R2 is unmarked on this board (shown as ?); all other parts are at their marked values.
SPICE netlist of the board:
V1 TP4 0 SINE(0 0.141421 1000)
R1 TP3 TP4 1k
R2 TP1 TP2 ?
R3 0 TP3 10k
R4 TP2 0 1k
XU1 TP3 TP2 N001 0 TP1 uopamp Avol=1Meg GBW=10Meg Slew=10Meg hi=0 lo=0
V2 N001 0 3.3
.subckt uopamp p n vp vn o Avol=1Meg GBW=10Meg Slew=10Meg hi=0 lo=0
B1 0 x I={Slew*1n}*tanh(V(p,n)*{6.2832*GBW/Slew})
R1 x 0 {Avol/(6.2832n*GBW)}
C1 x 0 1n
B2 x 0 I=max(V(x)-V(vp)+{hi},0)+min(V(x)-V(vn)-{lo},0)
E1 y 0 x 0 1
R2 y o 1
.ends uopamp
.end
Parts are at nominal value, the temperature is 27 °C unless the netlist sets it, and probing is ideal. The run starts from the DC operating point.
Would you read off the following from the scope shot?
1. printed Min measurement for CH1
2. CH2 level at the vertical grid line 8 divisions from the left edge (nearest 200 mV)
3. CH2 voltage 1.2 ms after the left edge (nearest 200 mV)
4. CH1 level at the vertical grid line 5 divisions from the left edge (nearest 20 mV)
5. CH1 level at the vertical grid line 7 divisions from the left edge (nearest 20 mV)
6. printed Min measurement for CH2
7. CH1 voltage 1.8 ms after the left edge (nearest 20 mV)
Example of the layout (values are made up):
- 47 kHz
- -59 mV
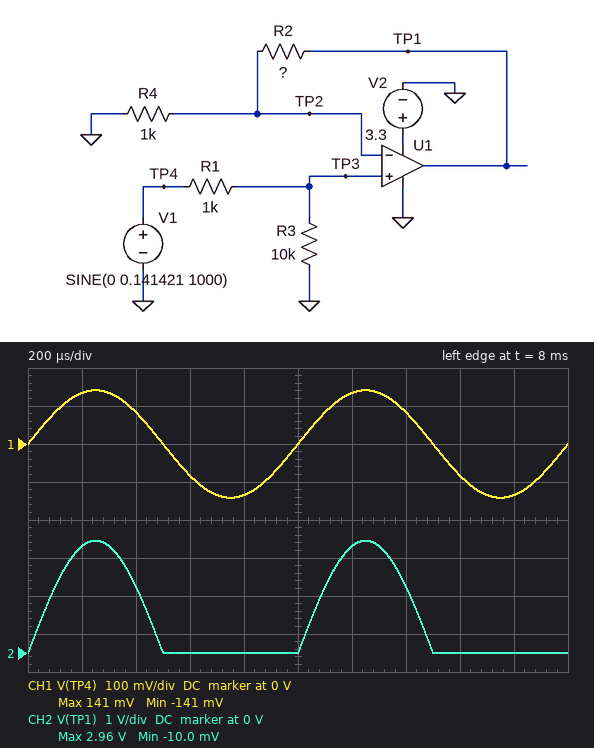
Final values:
- -141 mV
- 0 V
- 2.8 V
- 0 V
- 80 mV
- -10.0 mV
- -140 mV
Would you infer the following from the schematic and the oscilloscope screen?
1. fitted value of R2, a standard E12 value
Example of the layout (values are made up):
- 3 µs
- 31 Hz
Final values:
- 22 kΩ
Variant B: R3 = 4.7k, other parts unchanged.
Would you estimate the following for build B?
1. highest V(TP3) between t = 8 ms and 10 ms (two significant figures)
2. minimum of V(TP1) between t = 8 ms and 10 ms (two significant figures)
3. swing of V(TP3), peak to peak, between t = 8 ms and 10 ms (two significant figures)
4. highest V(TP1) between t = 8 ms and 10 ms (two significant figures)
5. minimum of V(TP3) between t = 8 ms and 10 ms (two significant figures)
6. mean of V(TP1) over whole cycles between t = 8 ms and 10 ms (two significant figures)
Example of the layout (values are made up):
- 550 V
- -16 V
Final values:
- 120 mV
- -6.2 mV
- 230 mV
- 2.7 V
- -120 mV
- 850 mV
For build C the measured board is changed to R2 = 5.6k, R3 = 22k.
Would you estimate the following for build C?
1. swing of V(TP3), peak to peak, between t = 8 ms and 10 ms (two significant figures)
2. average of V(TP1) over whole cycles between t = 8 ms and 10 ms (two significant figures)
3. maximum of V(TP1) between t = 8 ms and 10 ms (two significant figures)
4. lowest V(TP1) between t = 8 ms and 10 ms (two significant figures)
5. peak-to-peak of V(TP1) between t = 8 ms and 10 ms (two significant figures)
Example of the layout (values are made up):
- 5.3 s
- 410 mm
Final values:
- 270 mV
- 280 mV
- 890 mV
- -6.9 mV
- 900 mV
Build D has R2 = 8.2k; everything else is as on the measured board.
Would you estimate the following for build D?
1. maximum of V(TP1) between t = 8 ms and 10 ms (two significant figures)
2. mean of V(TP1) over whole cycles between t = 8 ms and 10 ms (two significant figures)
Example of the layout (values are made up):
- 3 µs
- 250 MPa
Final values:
- 1.2 V
- 370 mV
